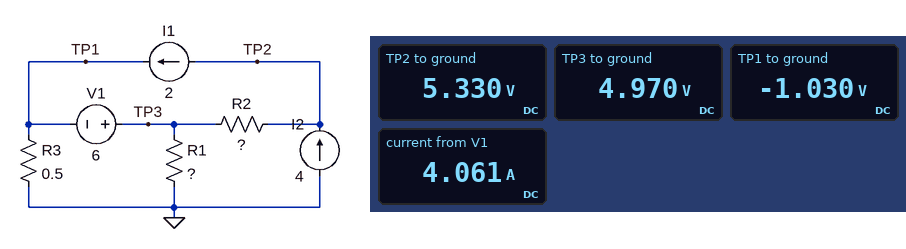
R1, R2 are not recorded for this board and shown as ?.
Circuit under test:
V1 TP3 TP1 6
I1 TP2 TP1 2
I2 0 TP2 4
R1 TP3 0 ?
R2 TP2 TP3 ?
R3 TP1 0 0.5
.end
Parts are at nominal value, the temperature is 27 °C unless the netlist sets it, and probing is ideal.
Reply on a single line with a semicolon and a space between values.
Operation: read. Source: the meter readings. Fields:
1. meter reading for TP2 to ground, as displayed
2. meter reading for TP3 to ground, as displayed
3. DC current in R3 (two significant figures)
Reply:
5.330 V; 4.970 V; 2.1 A
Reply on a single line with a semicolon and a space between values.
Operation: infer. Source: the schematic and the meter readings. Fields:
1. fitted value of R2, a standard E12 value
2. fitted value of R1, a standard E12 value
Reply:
0.18 Ω; 0.82 Ω
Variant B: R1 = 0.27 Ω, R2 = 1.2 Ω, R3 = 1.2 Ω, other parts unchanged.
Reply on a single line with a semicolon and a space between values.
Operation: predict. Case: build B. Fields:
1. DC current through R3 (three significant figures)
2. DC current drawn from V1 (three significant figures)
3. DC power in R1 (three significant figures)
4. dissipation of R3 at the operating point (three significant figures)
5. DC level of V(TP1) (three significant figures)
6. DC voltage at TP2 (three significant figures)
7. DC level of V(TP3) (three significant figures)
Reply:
3.35 A; 5.35 A; 14.6 W; 13.4 W; -4.02 V; 4.38 V; 1.98 V
